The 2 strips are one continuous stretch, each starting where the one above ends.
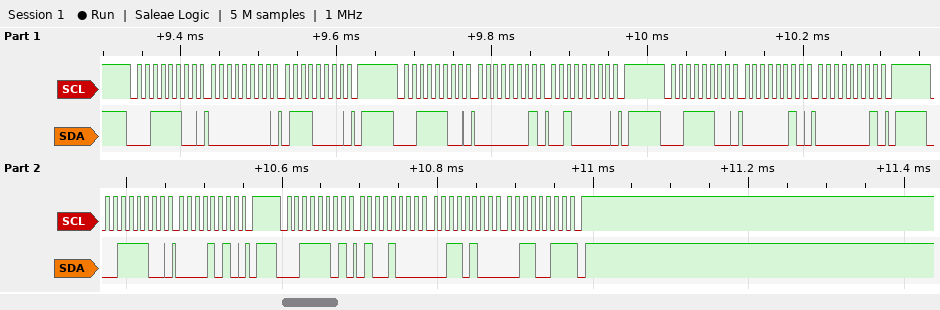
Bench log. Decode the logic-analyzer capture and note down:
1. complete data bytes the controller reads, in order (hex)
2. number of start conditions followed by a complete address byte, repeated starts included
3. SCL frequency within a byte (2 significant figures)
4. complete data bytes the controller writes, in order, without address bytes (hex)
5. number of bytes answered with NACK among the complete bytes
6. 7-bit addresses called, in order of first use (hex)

48 34 33
5
100 kHz
00 70 01 20 02 01 0A
1
0x1E
